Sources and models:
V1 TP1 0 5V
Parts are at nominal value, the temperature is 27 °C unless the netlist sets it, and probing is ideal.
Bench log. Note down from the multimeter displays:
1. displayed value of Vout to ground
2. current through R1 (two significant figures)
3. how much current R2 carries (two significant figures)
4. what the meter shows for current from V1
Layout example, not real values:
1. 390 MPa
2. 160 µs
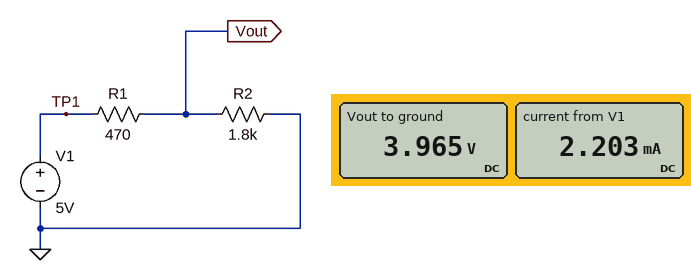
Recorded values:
1. 3.965 V
2. 2.2 mA
3. 2.2 mA
4. 2.203 mA
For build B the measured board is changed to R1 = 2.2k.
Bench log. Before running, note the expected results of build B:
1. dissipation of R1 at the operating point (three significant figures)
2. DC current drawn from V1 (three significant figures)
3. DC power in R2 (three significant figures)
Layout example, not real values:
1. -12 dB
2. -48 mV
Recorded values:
1. 3.44 mW
2. 1.25 mA
3. 2.81 mW
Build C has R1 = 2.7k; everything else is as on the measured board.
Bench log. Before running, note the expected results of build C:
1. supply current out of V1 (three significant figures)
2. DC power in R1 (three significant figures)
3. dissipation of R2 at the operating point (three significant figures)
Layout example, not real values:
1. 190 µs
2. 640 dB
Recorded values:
1. 1.11 mA
2. 3.33 mW
3. 2.22 mW
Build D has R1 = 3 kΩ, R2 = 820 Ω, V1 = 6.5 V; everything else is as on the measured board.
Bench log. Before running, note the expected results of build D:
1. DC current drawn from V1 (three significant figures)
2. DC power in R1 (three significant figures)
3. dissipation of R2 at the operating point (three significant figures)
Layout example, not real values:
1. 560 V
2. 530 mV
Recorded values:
1. 1.70 mA
2. 8.69 mW
3. 2.37 mW
